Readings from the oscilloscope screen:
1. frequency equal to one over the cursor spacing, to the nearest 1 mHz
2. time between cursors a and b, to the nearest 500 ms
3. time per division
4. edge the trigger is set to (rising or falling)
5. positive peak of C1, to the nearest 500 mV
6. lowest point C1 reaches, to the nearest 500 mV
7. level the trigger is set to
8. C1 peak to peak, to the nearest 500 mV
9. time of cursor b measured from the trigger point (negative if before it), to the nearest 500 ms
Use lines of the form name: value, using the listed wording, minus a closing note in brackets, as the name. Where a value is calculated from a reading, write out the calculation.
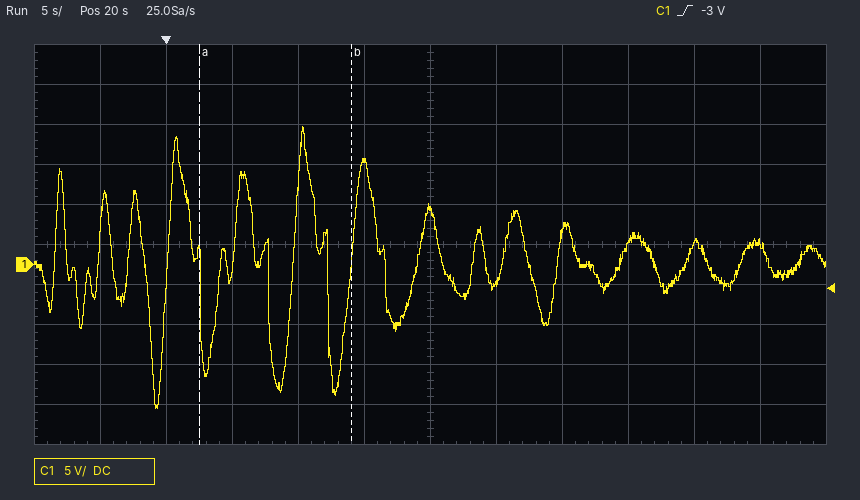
frequency equal to one over the cursor spacing, to the nearest 1 mHz: 1 / 11.5 s ≈ 87 mHz
time between cursors a and b, to the nearest 500 ms: 11.5 s
time per division: 5 s
edge the trigger is set to: rising
positive peak of C1, to the nearest 500 mV: 17.0 V
lowest point C1 reaches, to the nearest 500 mV: -18.0 V
level the trigger is set to: -3 V
C1 peak to peak, to the nearest 500 mV: 17.0 V − (-18.0 V) = 35.0 V
time of cursor b measured from the trigger point (negative if before it), to the nearest 500 ms: +14.0 s
